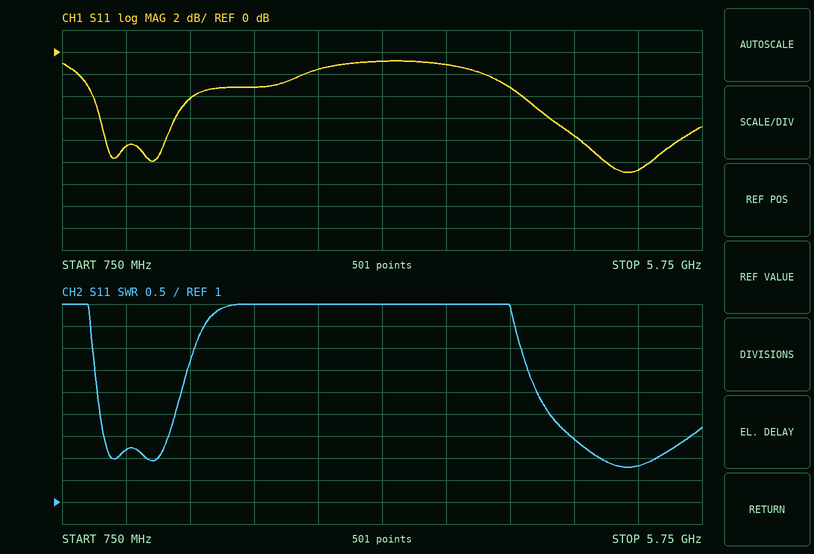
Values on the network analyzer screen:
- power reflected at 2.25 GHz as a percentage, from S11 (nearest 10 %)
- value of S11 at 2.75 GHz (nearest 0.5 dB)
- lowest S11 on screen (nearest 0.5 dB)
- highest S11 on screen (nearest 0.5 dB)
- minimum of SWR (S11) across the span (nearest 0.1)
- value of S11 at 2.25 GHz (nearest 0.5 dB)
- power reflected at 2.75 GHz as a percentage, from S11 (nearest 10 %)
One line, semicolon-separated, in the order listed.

50 %; -1.5 dB; -11.0 dB; -1.0 dB; 1.8; -3.0 dB; 70 %
